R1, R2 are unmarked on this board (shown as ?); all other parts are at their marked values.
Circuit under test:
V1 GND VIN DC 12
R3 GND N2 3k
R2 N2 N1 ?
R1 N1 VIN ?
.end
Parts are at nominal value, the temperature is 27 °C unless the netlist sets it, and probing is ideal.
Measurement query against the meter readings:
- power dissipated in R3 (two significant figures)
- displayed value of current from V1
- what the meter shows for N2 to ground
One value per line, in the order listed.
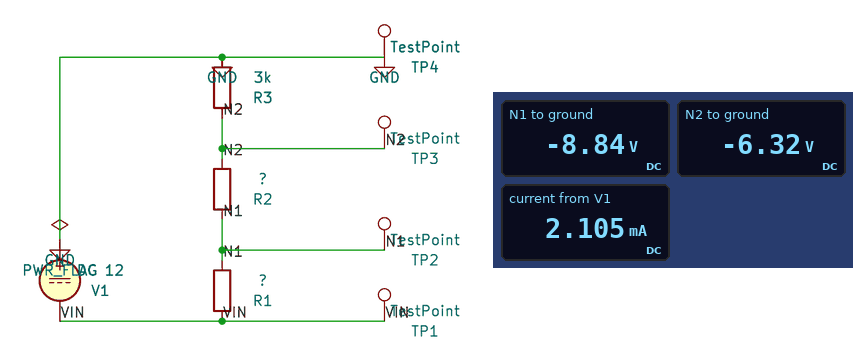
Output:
13 mW
2.105 mA
-6.32 V
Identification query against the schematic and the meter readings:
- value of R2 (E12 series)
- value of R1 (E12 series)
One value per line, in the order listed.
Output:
1.2 kΩ
1.5 kΩ
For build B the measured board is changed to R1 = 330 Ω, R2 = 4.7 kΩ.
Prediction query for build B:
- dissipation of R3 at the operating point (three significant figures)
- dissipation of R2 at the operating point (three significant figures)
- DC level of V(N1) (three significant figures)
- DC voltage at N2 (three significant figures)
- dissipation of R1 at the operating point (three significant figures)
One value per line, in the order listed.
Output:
6.70 mW
10.5 mW
-11.5 V
-4.48 V
737 µW
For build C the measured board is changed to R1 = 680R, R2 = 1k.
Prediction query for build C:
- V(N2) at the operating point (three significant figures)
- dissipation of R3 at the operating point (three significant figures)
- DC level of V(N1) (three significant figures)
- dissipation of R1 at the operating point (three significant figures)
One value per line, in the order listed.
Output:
-7.69 V
19.7 mW
-10.3 V
4.47 mW
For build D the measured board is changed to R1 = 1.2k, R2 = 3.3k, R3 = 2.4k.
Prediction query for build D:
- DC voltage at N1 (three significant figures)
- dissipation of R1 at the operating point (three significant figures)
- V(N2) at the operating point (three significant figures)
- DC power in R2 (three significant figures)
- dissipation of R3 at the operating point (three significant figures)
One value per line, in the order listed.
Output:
-9.91 V
3.63 mW
-4.17 V
9.98 mW
7.26 mW
